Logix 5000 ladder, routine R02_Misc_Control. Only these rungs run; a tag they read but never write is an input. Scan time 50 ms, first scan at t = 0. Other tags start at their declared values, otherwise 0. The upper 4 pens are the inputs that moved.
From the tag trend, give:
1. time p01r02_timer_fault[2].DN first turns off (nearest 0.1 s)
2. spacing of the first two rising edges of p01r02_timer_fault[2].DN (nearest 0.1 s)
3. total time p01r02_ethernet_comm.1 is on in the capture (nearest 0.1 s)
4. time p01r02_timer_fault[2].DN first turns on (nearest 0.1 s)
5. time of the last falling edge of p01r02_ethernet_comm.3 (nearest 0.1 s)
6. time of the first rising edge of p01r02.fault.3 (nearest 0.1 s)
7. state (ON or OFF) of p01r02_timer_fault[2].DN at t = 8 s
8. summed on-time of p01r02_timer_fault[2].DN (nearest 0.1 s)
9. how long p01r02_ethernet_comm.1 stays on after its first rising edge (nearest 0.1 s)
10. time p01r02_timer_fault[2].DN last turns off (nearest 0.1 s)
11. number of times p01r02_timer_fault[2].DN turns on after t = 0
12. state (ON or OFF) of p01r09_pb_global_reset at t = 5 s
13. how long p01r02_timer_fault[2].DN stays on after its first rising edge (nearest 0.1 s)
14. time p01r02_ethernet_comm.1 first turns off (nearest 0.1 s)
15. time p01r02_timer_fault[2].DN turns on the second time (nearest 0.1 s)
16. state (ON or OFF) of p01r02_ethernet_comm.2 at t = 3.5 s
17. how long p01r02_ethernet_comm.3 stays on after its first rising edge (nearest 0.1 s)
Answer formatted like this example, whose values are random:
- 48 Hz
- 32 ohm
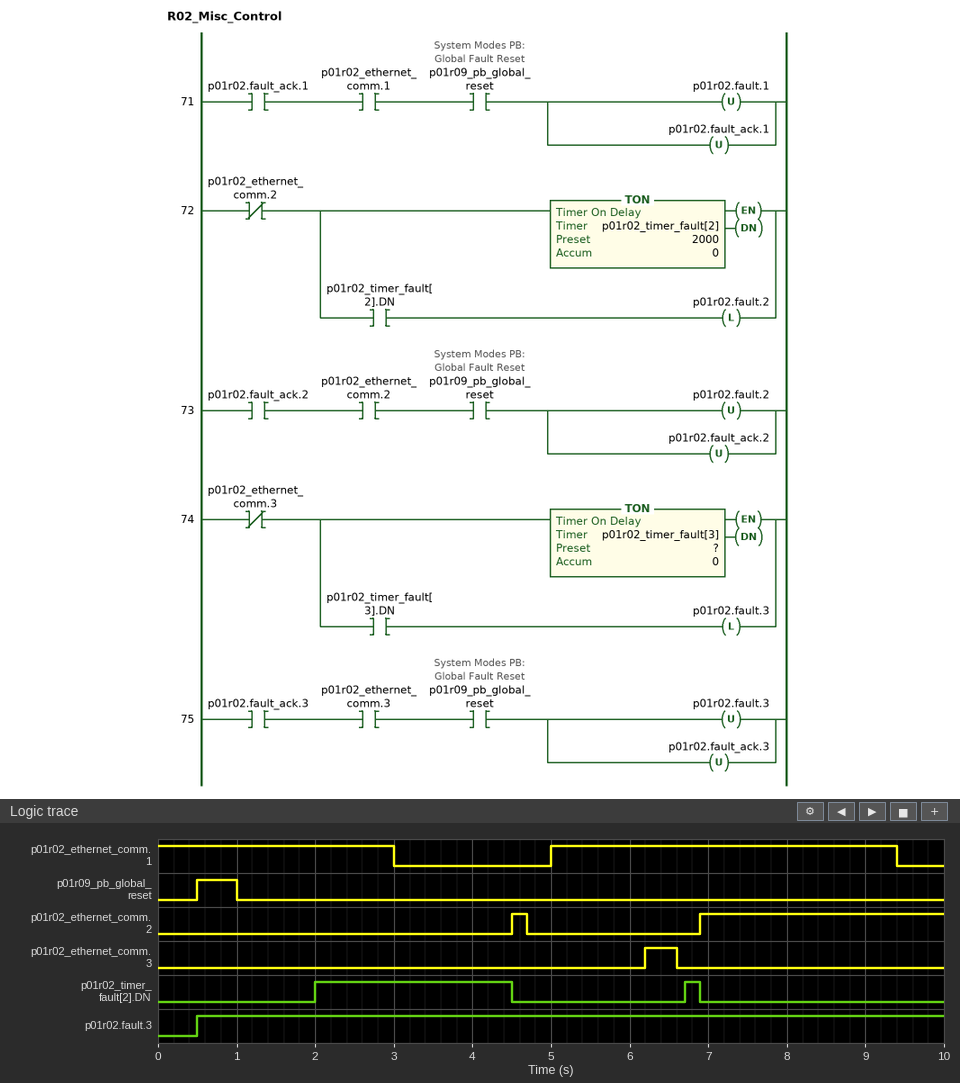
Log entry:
- 4.5 s
- 4.7 s
- 7.4 s
- 2.0 s
- 6.6 s
- 0.5 s
- OFF
- 2.7 s
- 4.4 s
- 6.9 s
- 2
- OFF
- 2.5 s
- 3.0 s
- 6.7 s
- OFF
- 0.4 s
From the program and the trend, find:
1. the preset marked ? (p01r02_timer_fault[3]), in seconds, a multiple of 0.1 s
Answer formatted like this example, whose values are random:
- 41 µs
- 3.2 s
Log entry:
- 0.5 s
